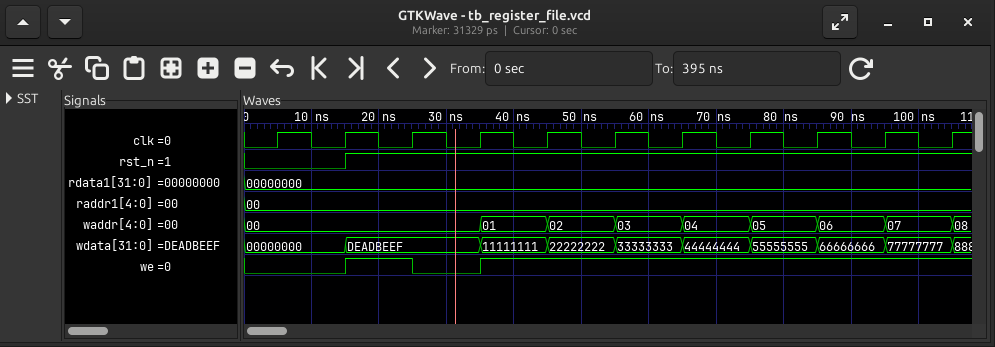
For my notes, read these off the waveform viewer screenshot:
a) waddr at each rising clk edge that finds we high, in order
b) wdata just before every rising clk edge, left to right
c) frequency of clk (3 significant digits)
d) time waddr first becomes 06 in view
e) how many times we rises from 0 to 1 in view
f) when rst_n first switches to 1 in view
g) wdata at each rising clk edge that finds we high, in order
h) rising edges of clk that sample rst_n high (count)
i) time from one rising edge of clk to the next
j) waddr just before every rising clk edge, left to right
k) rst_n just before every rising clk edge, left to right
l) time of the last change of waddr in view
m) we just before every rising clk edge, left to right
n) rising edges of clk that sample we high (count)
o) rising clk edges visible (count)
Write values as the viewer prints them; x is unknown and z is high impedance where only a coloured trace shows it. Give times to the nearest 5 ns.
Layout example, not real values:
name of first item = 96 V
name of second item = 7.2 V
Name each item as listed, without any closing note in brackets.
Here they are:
waddr at each rising clk edge that finds we high, in order = 00, 01, 02, 03, 04, 05, 06, 07
wdata just before every rising clk edge, left to right = 00000000, 00000000, DEADBEEF, DEADBEEF, 11111111, 22222222, 33333333, 44444444, 55555555, 66666666, 77777777
frequency of clk = 100 MHz
time waddr first becomes 06 in view = 85 ns
how many times we rises from 0 to 1 in view = 2
when rst_n first switches to 1 in view = 15 ns
wdata at each rising clk edge that finds we high, in order = DEADBEEF, 11111111, 22222222, 33333333, 44444444, 55555555, 66666666, 77777777
rising edges of clk that sample rst_n high = 9
time from one rising edge of clk to the next = 10 ns
waddr just before every rising clk edge, left to right = 00, 00, 00, 00, 01, 02, 03, 04, 05, 06, 07
rst_n just before every rising clk edge, left to right = 0 0 1 1 1 1 1 1 1 1 1
time of the last change of waddr in view = 105 ns
we just before every rising clk edge, left to right = 0 0 1 0 1 1 1 1 1 1 1
rising edges of clk that sample we high = 8
rising clk edges visible = 11
